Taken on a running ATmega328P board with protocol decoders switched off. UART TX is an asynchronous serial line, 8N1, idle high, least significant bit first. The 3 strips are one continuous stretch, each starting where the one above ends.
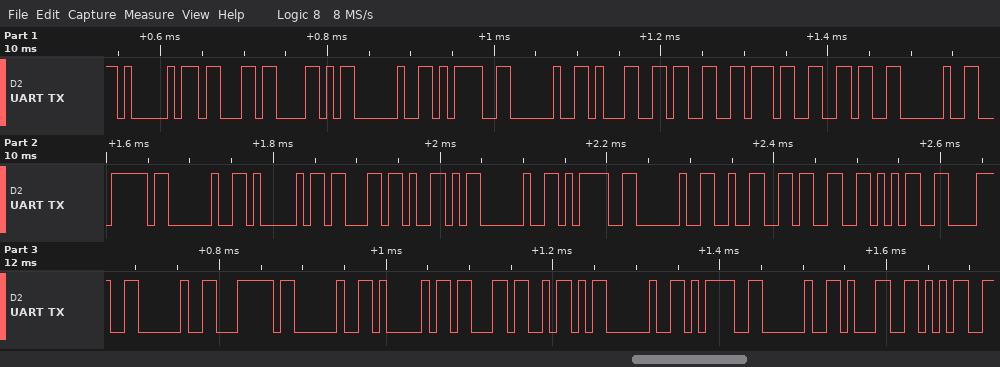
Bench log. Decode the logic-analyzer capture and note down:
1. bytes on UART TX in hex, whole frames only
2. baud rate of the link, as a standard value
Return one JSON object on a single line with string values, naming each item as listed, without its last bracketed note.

{"bytes on UART TX in hex, whole frames only": "41 63 58 20 3D 20 31 33 37 36 20 7C 20 41 63 59 20 3D 20 32 33 35 38 20 7C 20 41 63 5A 20 3D 20 31 35", "baud rate of the link, as a standard value": "115200 baud"}
